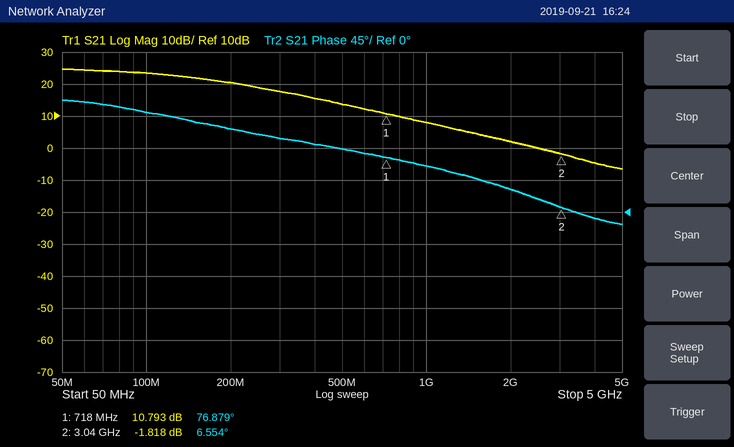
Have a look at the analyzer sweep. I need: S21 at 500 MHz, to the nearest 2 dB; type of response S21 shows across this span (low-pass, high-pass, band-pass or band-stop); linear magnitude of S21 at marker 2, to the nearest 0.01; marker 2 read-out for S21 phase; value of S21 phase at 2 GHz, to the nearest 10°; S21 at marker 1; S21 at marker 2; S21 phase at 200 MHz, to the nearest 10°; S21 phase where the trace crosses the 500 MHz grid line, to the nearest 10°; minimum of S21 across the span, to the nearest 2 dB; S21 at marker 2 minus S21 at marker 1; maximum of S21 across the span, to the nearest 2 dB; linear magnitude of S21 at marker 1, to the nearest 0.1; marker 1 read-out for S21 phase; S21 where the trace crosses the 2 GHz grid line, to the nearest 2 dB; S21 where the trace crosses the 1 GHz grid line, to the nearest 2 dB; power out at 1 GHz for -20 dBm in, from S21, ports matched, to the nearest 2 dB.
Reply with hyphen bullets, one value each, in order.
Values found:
- 14 dB
- low-pass
- 0.81
- 6.554°
- 30°
- 10.793 dB
- -1.818 dB
- 120°
- 90°
- -6 dB
- -12.611 dB
- 24 dB
- 3.5
- 76.879°
- 2 dB
- 8 dB
- -12 dBm
